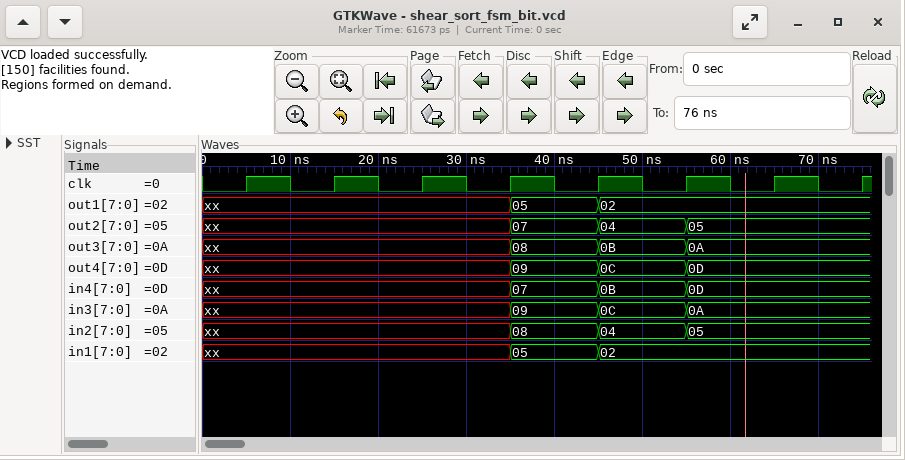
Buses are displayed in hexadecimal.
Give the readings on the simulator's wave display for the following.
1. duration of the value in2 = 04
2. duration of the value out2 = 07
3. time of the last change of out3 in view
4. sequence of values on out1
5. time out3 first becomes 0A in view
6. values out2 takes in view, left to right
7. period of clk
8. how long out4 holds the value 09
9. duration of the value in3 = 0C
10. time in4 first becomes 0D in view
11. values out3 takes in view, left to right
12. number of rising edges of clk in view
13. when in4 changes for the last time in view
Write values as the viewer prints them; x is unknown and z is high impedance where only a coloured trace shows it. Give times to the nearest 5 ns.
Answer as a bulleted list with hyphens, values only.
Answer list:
- 10 ns
- 10 ns
- 55 ns
- xx, 05, 02
- 55 ns
- xx, 07, 04, 05
- 10 ns
- 10 ns
- 10 ns
- 55 ns
- xx, 08, 0B, 0A
- 8
- 55 ns
